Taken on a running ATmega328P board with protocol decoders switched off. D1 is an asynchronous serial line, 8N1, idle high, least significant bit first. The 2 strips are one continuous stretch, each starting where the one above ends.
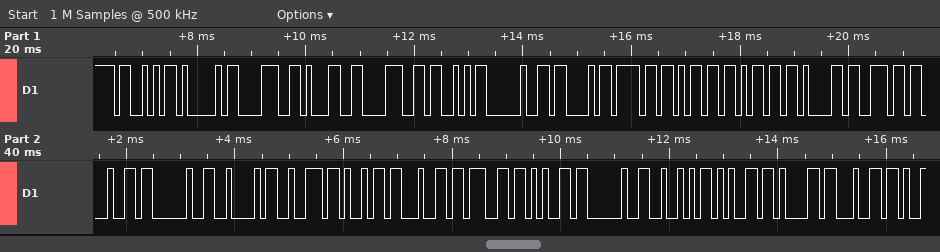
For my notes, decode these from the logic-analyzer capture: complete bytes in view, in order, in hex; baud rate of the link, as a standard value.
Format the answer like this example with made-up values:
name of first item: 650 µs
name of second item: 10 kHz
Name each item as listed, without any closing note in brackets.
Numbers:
complete bytes in view, in order, in hex: 0x53 0x41 0x38 0x31 0x38 0x53 0x20 0x43 0x6F 0x6D 0x6D 0x61 0x6E 0x64 0x20 0x42 0x72 0x69 0x64 0x67 0x65 0x20 0x52 0x65 0x61 0x64
baud rate of the link, as a standard value: 9600 baud
